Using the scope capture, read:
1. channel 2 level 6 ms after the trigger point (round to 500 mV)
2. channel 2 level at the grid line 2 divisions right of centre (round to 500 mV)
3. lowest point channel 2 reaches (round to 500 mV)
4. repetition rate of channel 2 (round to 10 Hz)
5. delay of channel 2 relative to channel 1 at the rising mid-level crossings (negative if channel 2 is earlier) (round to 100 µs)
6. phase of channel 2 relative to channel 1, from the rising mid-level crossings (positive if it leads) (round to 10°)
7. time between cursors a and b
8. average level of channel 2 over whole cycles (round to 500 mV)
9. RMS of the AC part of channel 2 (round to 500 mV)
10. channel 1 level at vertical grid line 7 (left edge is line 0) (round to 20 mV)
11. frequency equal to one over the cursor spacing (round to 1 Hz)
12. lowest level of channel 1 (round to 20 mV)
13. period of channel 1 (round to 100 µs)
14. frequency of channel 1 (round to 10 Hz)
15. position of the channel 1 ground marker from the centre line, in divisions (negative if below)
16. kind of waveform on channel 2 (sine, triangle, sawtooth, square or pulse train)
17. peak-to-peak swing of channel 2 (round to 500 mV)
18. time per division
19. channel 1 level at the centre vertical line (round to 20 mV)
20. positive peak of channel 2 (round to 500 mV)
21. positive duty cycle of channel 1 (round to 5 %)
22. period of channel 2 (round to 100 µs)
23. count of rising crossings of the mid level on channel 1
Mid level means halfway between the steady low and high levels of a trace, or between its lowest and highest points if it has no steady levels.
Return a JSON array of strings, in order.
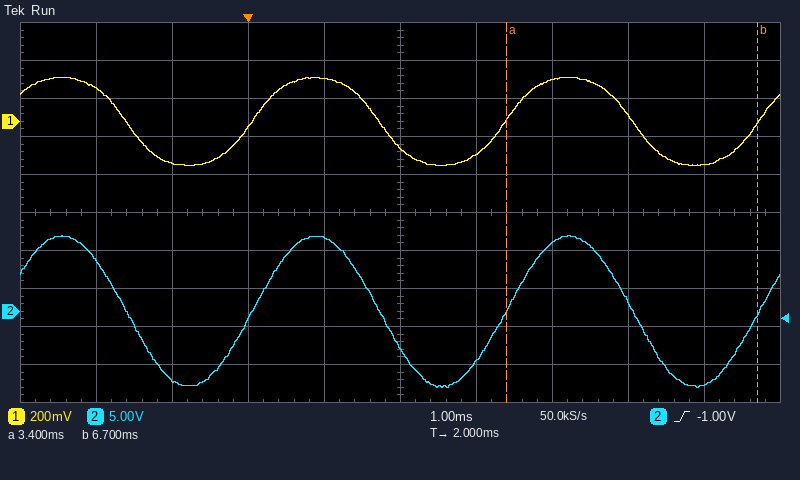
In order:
["-9.5 V", "9.0 V", "-10.0 V", "300 Hz", "0.0 ms", "0°", "3.3 ms", "0.0 V", "7.0 V", "220 mV", "303 Hz", "-240 mV", "3.3 ms", "300 Hz", "+2.4 div", "sine", "20.0 V", "1 ms", "-140 mV", "10.0 V", "50 %", "3.3 ms", "3"]
